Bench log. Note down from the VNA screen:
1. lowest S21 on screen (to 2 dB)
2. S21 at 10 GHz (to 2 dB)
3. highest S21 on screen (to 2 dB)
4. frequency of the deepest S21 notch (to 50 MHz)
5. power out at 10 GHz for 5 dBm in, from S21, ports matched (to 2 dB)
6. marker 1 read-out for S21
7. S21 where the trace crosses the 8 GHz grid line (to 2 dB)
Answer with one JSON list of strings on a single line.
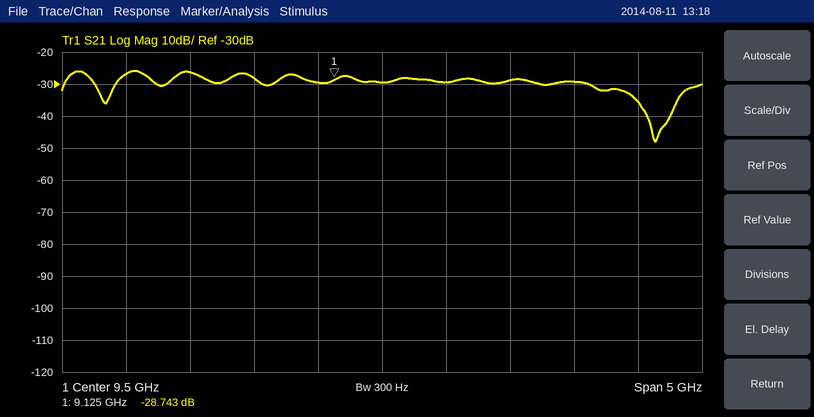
["-48 dB", "-30 dB", "-26 dB", "11.65 GHz", "-24 dBm", "-28.743 dB", "-26 dB"]
